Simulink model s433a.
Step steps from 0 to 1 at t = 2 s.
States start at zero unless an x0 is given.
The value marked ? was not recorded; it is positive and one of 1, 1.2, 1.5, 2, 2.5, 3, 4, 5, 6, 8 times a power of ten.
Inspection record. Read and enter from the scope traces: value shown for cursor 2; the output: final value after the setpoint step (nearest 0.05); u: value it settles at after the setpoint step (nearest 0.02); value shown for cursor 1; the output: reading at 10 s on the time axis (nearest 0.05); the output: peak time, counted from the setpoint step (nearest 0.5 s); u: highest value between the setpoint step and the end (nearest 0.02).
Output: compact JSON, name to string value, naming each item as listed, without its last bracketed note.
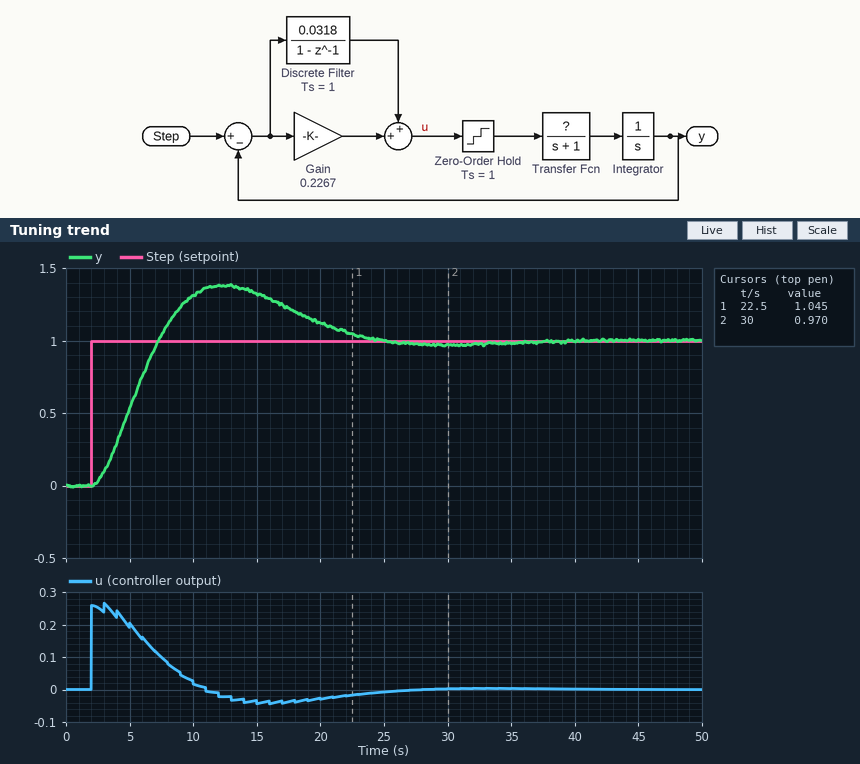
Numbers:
{"value shown for cursor 2": "0.970", "the output: final value after the setpoint step": "1.00", "u: value it settles at after the setpoint step": "0.00", "value shown for cursor 1": "1.045", "the output: reading at 10 s on the time axis": "1.30", "the output: peak time, counted from the setpoint step": "10.5 s", "u: highest value between the setpoint step and the end": "0.26"}
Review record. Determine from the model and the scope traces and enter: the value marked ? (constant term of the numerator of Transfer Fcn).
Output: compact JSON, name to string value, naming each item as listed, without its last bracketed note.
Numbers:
{"the value marked ?": "1"}
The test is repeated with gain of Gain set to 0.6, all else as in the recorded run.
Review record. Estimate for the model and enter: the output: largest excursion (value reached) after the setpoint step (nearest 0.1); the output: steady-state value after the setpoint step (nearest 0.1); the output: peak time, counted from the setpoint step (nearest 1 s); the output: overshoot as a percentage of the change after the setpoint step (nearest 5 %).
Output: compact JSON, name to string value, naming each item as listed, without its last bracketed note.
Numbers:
{"the output: largest excursion (value reached) after the setpoint step": "1.3", "the output: steady-state value after the setpoint step": "1.0", "the output: peak time, counted from the setpoint step": "5 s", "the output: overshoot as a percentage of the change after the setpoint step": "35 %"}
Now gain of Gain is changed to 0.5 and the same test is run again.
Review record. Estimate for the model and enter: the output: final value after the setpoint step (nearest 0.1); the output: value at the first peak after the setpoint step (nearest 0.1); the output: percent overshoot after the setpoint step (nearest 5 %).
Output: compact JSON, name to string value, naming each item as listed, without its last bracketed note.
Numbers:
{"the output: final value after the setpoint step": "1.0", "the output: value at the first peak after the setpoint step": "1.3", "the output: percent overshoot after the setpoint step": "30 %"}
